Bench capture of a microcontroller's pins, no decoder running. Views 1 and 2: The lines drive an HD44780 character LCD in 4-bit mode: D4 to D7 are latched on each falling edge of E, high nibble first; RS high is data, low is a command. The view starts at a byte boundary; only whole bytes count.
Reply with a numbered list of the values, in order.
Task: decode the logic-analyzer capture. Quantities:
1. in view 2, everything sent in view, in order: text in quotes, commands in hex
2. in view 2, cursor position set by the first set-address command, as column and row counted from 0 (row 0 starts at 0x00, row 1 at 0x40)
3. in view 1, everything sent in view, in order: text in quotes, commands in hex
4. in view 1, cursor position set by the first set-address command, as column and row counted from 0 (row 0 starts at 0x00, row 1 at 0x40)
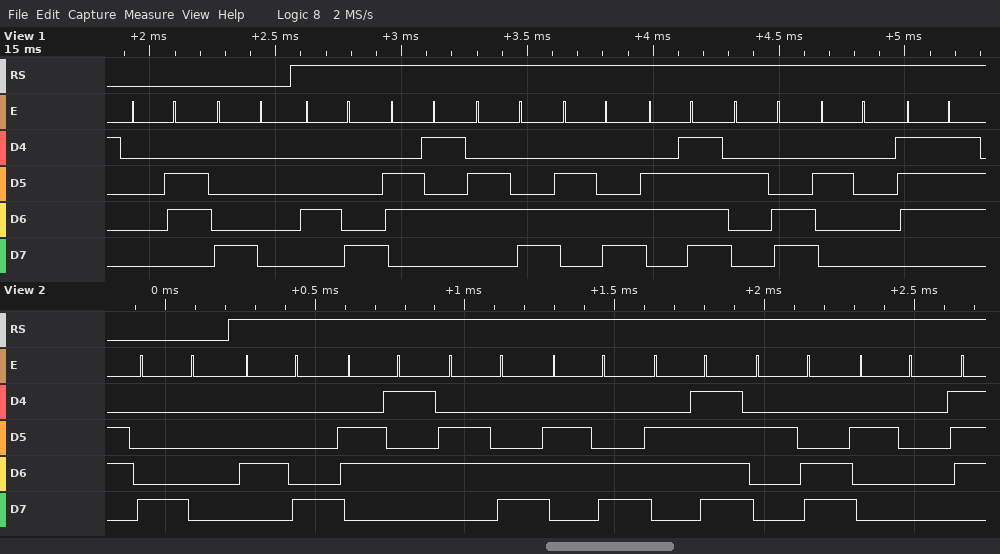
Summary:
1. 0x80 "Hello, "
2. column 0, row 0
3. 0x06 0x80 "Hello, w"
4. column 0, row 0
